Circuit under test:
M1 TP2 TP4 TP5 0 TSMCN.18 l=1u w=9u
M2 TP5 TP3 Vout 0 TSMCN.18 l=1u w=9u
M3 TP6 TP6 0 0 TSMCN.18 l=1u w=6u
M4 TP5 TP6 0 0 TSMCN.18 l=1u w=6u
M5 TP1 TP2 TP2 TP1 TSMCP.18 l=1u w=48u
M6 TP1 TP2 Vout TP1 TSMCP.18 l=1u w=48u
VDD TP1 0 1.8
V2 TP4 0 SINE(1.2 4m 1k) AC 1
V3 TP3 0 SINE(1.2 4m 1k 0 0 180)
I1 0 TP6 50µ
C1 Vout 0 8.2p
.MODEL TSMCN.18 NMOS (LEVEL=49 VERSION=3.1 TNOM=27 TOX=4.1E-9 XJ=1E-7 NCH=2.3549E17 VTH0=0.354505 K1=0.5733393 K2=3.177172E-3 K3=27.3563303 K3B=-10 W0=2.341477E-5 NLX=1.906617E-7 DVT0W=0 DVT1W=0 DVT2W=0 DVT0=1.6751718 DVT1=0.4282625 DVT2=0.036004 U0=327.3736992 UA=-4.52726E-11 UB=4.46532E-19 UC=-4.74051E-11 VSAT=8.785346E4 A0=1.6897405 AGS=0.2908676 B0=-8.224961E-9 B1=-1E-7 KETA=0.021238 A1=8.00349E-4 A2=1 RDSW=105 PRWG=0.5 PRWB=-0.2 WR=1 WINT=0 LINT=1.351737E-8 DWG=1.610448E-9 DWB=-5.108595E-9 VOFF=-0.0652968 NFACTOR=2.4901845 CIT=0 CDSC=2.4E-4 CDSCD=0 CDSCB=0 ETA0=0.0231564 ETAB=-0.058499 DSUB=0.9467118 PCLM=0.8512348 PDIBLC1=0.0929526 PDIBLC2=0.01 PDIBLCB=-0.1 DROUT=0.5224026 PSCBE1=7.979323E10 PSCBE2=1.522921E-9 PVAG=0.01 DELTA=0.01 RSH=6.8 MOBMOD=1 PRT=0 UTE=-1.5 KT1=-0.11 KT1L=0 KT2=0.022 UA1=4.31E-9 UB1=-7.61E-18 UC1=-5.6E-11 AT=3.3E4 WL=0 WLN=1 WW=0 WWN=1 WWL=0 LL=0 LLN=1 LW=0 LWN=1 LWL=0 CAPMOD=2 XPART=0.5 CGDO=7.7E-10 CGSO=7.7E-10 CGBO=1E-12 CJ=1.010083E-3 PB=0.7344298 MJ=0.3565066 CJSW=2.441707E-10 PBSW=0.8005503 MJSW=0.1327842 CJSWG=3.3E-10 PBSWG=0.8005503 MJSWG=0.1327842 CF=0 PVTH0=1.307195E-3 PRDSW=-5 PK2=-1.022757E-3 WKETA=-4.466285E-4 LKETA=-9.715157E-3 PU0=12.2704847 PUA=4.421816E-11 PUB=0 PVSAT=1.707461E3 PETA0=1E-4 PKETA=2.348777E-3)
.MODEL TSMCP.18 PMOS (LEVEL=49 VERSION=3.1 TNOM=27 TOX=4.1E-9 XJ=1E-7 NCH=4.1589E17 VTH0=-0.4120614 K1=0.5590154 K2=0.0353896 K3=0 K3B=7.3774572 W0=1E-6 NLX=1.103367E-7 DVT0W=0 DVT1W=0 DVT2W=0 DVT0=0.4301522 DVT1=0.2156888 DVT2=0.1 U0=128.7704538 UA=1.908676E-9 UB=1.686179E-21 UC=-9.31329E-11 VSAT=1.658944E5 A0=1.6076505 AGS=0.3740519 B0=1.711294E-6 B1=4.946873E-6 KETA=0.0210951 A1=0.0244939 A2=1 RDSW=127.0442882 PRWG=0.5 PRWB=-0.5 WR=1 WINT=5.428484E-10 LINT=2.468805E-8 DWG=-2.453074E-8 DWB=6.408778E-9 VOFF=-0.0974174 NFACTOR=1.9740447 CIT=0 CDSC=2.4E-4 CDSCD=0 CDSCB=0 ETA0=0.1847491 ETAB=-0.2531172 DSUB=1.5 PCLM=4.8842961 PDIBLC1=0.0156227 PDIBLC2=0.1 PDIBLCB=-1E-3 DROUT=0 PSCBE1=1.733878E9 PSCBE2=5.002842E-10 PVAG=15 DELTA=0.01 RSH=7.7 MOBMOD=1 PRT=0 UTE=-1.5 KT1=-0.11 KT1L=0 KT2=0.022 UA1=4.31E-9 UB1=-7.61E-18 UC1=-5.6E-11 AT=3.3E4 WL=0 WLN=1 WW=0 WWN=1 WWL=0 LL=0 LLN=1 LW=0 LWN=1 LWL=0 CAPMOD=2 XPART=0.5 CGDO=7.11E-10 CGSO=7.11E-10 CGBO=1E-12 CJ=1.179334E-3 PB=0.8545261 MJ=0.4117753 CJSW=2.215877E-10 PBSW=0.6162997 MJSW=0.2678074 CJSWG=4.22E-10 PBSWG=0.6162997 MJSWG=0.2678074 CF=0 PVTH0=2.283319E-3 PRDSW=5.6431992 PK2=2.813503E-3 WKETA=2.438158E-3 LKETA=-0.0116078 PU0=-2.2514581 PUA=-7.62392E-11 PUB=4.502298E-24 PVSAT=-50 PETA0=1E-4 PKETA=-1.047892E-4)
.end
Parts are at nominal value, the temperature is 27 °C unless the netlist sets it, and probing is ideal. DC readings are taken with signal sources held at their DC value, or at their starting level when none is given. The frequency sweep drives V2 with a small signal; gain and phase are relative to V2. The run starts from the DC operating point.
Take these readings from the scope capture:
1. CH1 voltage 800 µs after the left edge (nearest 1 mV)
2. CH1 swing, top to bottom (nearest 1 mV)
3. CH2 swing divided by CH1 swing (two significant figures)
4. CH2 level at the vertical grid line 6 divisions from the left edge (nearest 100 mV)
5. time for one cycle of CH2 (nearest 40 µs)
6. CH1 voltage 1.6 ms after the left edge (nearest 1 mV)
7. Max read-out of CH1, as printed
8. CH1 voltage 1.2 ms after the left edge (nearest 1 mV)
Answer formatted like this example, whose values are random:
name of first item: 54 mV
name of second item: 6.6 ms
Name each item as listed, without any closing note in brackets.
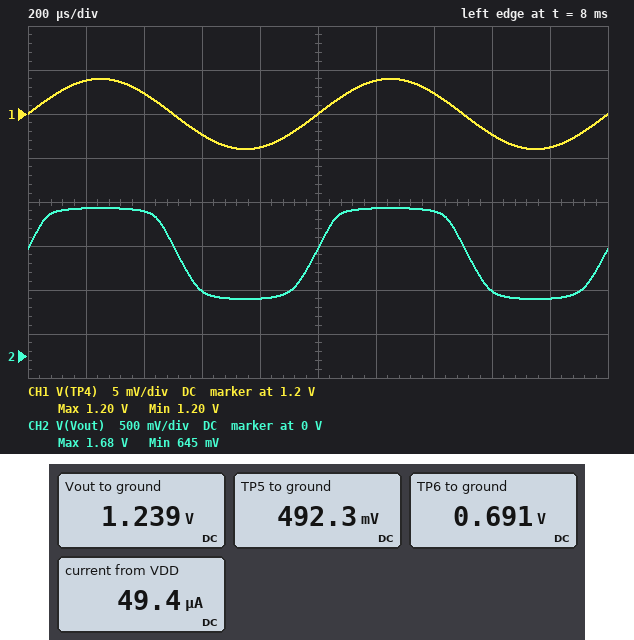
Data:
CH1 voltage 800 µs after the left edge: 1.196 V
CH1 swing, top to bottom: 8 mV
CH2 swing divided by CH1 swing: 130
CH2 level at the vertical grid line 6 divisions from the left edge: 1.7 V
time for one cycle of CH2: 1.00 ms
CH1 voltage 1.6 ms after the left edge: 1.198 V
Max read-out of CH1, as printed: 1.20 V
CH1 voltage 1.2 ms after the left edge: 1.204 V
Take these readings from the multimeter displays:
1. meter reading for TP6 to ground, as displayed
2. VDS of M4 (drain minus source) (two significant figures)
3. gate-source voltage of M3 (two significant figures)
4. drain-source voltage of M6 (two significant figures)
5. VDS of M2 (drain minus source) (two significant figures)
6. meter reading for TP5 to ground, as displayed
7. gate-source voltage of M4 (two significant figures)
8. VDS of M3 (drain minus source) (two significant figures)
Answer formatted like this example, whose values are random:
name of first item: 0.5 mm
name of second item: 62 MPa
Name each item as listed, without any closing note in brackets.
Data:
meter reading for TP6 to ground, as displayed: 0.691 V
VDS of M4 (drain minus source): 490 mV
gate-source voltage of M3: 690 mV
drain-source voltage of M6: 560 mV
VDS of M2 (drain minus source): -750 mV
meter reading for TP5 to ground, as displayed: 492.3 mV
gate-source voltage of M4: 690 mV
VDS of M3 (drain minus source): 690 mV
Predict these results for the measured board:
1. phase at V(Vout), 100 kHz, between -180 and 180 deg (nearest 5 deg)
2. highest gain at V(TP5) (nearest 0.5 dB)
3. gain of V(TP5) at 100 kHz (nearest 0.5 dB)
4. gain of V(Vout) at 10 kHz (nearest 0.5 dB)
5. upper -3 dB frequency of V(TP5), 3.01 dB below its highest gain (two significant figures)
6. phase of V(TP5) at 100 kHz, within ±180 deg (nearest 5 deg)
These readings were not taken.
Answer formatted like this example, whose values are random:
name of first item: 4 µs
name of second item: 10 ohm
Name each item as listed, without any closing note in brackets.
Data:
phase at V(Vout), 100 kHz, between -180 and 180 deg: -65 deg
highest gain at V(TP5): -3.5 dB
gain of V(TP5) at 100 kHz: -6.5 dB
gain of V(Vout) at 10 kHz: 42.0 dB
upper -3 dB frequency of V(TP5), 3.01 dB below its highest gain: 95 kHz
phase of V(TP5) at 100 kHz, within ±180 deg: -15 deg
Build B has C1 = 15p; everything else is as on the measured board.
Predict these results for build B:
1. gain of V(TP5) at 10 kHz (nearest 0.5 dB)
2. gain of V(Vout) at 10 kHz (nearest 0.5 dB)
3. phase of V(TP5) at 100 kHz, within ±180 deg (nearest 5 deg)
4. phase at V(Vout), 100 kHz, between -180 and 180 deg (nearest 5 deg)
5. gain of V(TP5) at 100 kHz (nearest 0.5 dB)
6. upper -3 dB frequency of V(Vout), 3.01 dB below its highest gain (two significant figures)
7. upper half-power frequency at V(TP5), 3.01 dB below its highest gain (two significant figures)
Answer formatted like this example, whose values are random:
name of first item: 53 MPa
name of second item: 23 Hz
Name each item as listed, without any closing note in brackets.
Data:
gain of V(TP5) at 10 kHz: -4.0 dB
gain of V(Vout) at 10 kHz: 41.5 dB
phase of V(TP5) at 100 kHz, within ±180 deg: -10 deg
phase at V(Vout), 100 kHz, between -180 and 180 deg: -75 deg
gain of V(TP5) at 100 kHz: -7.5 dB
upper -3 dB frequency of V(Vout), 3.01 dB below its highest gain: 28 kHz
upper half-power frequency at V(TP5), 3.01 dB below its highest gain: 52 kHz
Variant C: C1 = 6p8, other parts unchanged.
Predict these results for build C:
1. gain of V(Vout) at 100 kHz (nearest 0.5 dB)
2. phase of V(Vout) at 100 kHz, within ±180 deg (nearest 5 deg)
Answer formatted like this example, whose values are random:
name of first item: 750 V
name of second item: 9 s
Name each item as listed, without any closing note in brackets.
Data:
gain of V(Vout) at 100 kHz: 36.5 dB
phase of V(Vout) at 100 kHz, within ±180 deg: -60 deg
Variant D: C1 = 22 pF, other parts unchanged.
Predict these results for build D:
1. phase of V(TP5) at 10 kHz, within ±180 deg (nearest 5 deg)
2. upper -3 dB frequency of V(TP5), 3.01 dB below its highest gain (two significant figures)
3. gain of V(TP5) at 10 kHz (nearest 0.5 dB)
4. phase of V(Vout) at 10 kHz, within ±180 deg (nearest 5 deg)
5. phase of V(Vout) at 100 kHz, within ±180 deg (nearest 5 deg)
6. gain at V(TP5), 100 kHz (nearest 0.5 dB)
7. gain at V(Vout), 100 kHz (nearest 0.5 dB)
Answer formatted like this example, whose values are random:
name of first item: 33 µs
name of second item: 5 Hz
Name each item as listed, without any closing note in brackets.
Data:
phase of V(TP5) at 10 kHz, within ±180 deg: -10 deg
upper -3 dB frequency of V(TP5), 3.01 dB below its highest gain: 36 kHz
gain of V(TP5) at 10 kHz: -4.0 dB
phase of V(Vout) at 10 kHz, within ±180 deg: -30 deg
phase of V(Vout) at 100 kHz, within ±180 deg: -80 deg
gain at V(TP5), 100 kHz: -7.5 dB
gain at V(Vout), 100 kHz: 27.5 dB
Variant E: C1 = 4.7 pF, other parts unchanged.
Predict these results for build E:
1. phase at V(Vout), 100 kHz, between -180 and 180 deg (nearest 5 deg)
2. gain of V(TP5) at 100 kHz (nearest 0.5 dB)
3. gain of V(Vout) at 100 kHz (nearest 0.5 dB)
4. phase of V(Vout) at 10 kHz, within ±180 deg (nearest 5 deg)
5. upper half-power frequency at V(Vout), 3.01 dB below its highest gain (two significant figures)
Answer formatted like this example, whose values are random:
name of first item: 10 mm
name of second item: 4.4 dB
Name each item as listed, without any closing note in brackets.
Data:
phase at V(Vout), 100 kHz, between -180 and 180 deg: -50 deg
gain of V(TP5) at 100 kHz: -5.5 dB
gain of V(Vout) at 100 kHz: 38.5 dB
phase of V(Vout) at 10 kHz, within ±180 deg: -5 deg
upper half-power frequency at V(Vout), 3.01 dB below its highest gain: 87 kHz
